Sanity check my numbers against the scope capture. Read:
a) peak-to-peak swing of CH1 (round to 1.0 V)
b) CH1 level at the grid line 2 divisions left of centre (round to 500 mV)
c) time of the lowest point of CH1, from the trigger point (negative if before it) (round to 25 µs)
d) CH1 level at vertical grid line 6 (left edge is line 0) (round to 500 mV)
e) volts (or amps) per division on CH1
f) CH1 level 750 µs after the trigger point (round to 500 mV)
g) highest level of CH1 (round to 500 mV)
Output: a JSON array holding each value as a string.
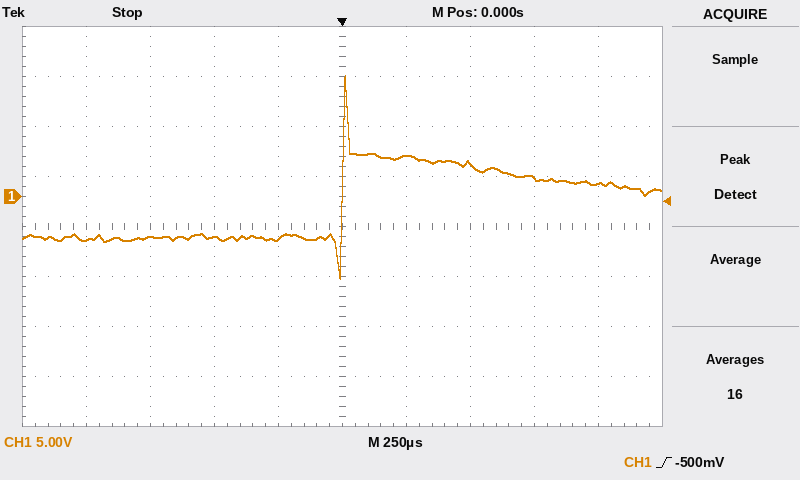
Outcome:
["20.0 V", "-4.0 V", "0 µs", "4.0 V", "5 V", "2.0 V", "12.0 V"]
